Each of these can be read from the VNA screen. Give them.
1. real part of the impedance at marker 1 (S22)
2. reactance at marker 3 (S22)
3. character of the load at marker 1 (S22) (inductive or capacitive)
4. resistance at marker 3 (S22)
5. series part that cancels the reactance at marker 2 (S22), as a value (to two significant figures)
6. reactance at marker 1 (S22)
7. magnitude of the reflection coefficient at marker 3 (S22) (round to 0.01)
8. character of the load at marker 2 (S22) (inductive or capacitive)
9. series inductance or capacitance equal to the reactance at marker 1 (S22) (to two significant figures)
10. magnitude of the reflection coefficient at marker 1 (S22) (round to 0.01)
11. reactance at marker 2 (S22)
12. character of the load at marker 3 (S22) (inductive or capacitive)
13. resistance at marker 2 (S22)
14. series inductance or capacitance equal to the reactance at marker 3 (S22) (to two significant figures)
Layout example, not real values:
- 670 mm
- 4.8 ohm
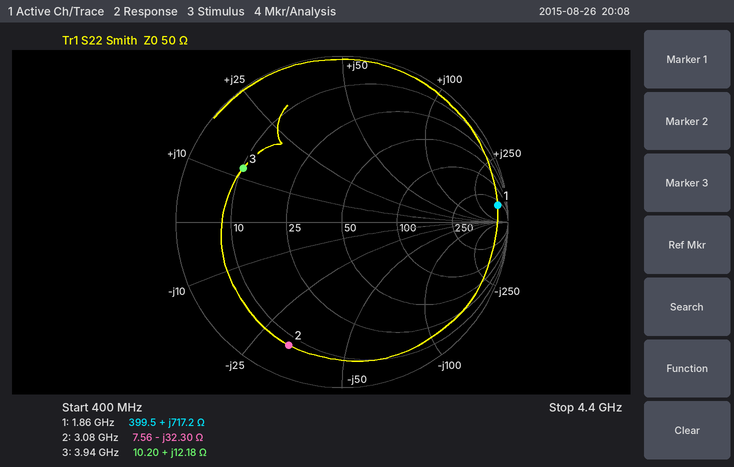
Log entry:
- 399.5 Ω
- +12.18 Ω
- inductive
- 10.20 Ω
- 1.7 nH
- +717.2 Ω
- 0.68
- capacitive
- 61 nH
- 0.94
- -32.30 Ω
- inductive
- 7.56 Ω
- 490 pH
